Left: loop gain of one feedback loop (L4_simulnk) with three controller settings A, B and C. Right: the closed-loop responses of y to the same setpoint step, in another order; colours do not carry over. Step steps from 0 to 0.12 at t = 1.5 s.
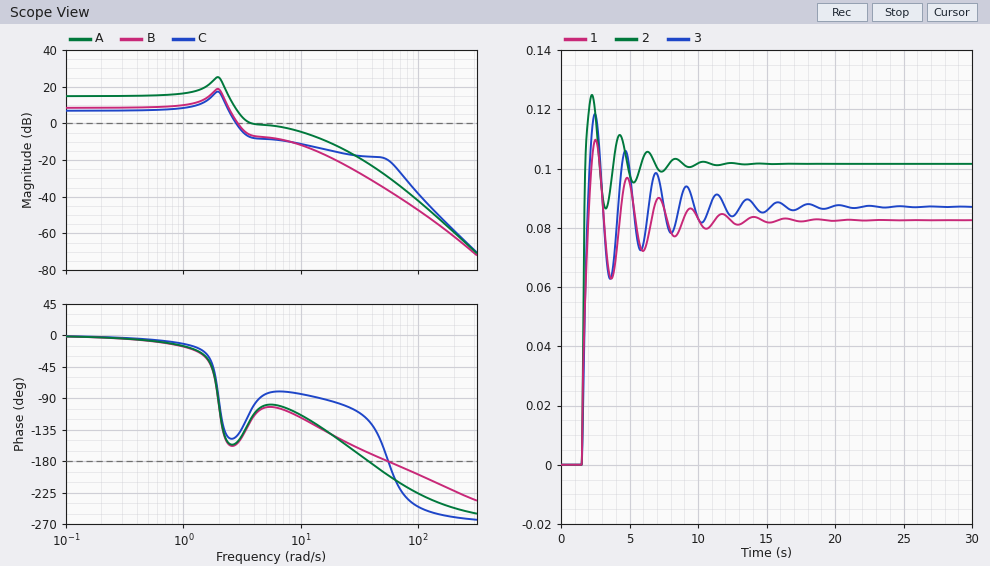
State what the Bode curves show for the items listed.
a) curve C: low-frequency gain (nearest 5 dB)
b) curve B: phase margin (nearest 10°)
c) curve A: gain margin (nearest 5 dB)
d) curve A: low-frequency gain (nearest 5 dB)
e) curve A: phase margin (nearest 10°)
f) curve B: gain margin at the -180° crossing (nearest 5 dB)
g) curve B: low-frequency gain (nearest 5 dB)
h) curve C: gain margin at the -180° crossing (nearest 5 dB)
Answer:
5 dB
30°
20 dB
15 dB
60°
35 dB
10 dB
20 dB
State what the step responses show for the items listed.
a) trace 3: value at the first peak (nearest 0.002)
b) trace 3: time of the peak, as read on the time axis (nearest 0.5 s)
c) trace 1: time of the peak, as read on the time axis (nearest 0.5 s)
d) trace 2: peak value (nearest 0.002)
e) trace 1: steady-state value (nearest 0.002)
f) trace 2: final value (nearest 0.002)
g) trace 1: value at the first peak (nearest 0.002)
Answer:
0.118
2.5 s
2.5 s
0.124
0.082
0.102
0.110
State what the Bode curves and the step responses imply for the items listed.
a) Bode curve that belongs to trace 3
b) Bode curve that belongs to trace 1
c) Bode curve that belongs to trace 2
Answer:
B
C
A
